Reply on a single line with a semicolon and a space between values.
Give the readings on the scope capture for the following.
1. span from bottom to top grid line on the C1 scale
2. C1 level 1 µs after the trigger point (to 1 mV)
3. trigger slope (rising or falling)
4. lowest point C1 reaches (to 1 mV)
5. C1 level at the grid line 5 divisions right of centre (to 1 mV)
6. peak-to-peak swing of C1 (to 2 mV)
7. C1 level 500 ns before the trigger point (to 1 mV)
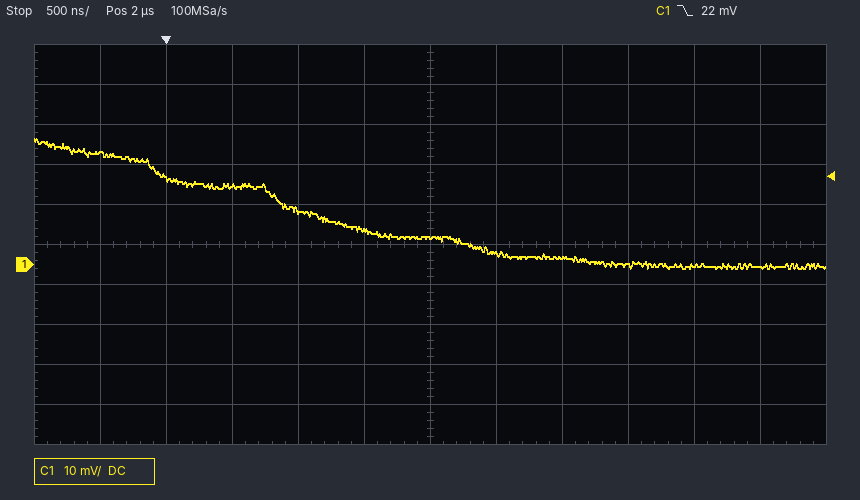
100 mV; 14 mV; falling; -1 mV; -1 mV; 32 mV; 28 mV
